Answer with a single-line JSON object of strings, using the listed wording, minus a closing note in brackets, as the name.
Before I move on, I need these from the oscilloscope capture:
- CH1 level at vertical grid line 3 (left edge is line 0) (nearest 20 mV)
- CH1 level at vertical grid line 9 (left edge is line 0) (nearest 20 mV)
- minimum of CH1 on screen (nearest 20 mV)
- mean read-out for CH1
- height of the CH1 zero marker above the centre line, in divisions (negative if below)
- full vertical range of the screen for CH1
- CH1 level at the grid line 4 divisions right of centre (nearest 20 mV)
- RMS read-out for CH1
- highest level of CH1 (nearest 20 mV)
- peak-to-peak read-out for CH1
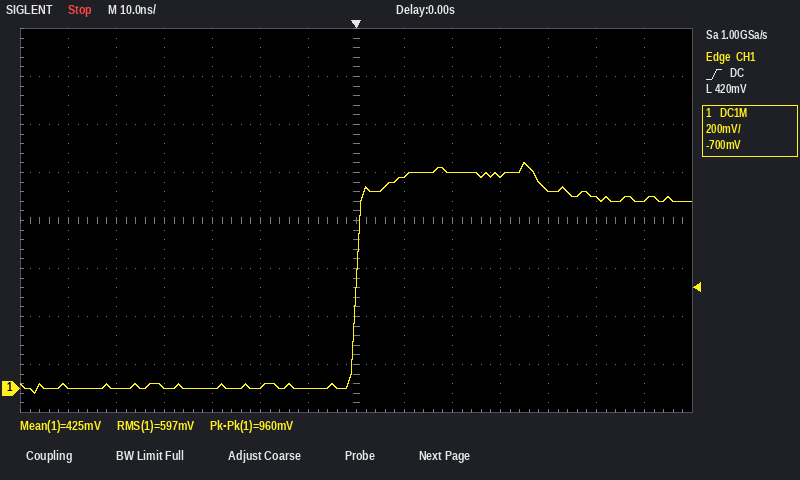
{"CH1 level at vertical grid line 3 (left edge is line 0)": "0 mV", "CH1 level at vertical grid line 9 (left edge is line 0)": "900 mV", "minimum of CH1 on screen": "-20 mV", "mean read-out for CH1": "425 mV", "height of the CH1 zero marker above the centre line, in divisions": "-3.5 div", "full vertical range of the screen for CH1": "1.6 V", "CH1 level at the grid line 4 divisions right of centre": "820 mV", "RMS read-out for CH1": "597 mV", "highest level of CH1": "940 mV", "peak-to-peak read-out for CH1": "960 mV"}
